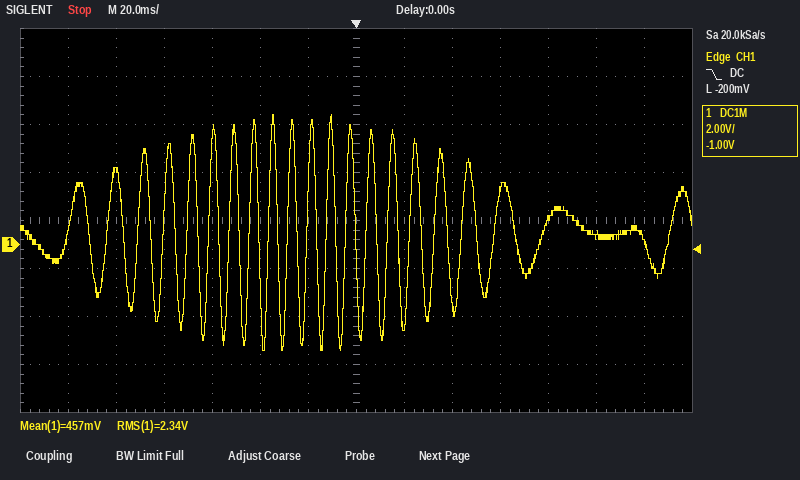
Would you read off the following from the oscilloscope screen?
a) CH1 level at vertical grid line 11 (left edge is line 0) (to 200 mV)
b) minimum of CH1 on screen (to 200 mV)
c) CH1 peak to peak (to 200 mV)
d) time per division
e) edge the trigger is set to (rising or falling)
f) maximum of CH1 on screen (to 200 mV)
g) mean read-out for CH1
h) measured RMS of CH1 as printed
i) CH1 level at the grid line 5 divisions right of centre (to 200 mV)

1.0 V
-4.4 V
9.8 V
20 ms
falling
5.4 V
457 mV
2.34 V
400 mV
